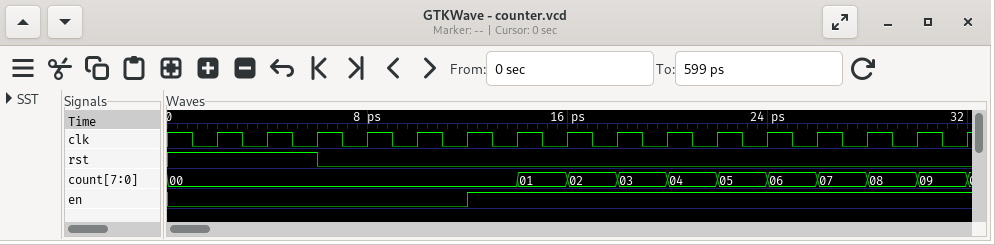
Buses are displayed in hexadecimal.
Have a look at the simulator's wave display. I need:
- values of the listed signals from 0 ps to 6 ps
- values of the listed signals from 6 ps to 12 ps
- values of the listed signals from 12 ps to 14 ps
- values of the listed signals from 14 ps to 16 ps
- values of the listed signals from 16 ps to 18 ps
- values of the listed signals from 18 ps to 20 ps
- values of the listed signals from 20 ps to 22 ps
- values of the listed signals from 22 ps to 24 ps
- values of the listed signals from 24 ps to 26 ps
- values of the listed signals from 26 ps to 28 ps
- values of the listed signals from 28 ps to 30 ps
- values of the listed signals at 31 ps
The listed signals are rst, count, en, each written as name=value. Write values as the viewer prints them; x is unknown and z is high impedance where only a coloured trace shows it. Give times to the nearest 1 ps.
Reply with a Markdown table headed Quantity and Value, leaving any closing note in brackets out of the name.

| Quantity | Value |
|---|---|
| values of the listed signals from 0 ps to 6 ps | rst=1, count=00, en=0 |
| values of the listed signals from 6 ps to 12 ps | rst=0, count=00, en=0 |
| values of the listed signals from 12 ps to 14 ps | rst=0, count=00, en=1 |
| values of the listed signals from 14 ps to 16 ps | rst=0, count=01, en=1 |
| values of the listed signals from 16 ps to 18 ps | rst=0, count=02, en=1 |
| values of the listed signals from 18 ps to 20 ps | rst=0, count=03, en=1 |
| values of the listed signals from 20 ps to 22 ps | rst=0, count=04, en=1 |
| values of the listed signals from 22 ps to 24 ps | rst=0, count=05, en=1 |
| values of the listed signals from 24 ps to 26 ps | rst=0, count=06, en=1 |
| values of the listed signals from 26 ps to 28 ps | rst=0, count=07, en=1 |
| values of the listed signals from 28 ps to 30 ps | rst=0, count=08, en=1 |
| values of the listed signals at 31 ps | rst=0, count=09, en=1 |
